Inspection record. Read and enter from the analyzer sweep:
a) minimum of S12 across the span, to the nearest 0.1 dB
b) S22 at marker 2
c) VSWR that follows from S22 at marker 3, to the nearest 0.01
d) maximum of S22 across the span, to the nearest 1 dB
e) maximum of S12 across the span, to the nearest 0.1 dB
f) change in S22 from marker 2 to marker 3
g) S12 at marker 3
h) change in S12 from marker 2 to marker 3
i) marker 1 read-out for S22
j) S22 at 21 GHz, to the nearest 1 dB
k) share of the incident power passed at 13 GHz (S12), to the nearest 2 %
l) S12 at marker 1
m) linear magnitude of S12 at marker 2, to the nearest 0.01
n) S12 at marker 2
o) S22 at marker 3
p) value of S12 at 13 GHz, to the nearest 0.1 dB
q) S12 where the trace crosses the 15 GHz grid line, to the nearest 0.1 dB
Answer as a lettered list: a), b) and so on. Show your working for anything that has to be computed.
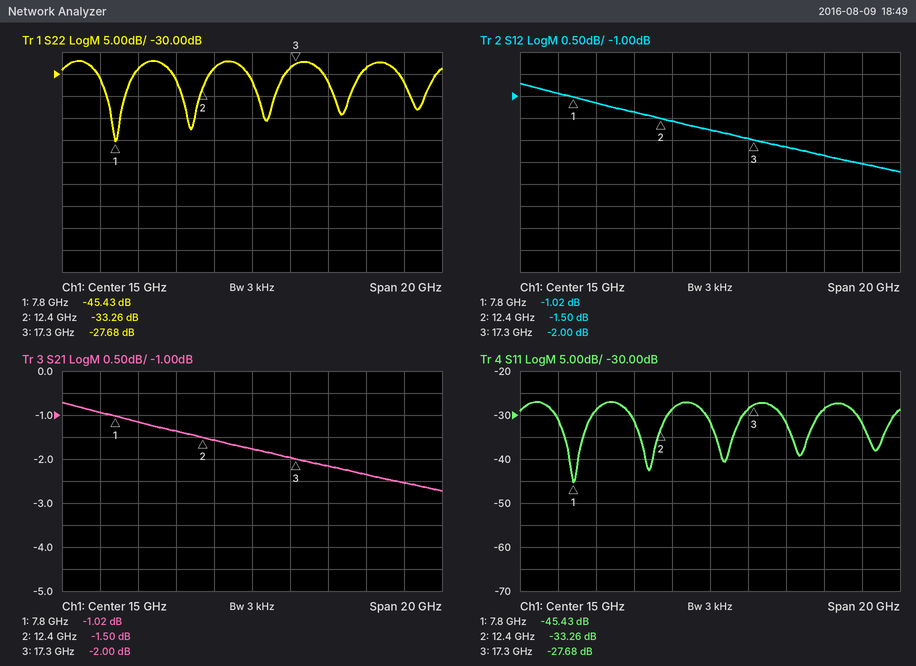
a) -2.7 dB
b) -33.26 dB
c) (1 + 0.0413)/(1 − 0.0413) ≈ 1.09
d) -27 dB
e) -0.7 dB
f) -27.68 − (-33.26) = 5.58 dB
g) -2.00 dB
h) -2 − (-1.5) = -0.50 dB
i) -45.43 dB
j) -29 dB
k) 10^(-1.6/10) ≈ 69.2 %, so 70 % to the nearest 2 %
l) -1.02 dB
m) 10^(-1.5/20) ≈ 0.84
n) -1.50 dB
o) -27.68 dB
p) -1.6 dB
q) -1.8 dB
